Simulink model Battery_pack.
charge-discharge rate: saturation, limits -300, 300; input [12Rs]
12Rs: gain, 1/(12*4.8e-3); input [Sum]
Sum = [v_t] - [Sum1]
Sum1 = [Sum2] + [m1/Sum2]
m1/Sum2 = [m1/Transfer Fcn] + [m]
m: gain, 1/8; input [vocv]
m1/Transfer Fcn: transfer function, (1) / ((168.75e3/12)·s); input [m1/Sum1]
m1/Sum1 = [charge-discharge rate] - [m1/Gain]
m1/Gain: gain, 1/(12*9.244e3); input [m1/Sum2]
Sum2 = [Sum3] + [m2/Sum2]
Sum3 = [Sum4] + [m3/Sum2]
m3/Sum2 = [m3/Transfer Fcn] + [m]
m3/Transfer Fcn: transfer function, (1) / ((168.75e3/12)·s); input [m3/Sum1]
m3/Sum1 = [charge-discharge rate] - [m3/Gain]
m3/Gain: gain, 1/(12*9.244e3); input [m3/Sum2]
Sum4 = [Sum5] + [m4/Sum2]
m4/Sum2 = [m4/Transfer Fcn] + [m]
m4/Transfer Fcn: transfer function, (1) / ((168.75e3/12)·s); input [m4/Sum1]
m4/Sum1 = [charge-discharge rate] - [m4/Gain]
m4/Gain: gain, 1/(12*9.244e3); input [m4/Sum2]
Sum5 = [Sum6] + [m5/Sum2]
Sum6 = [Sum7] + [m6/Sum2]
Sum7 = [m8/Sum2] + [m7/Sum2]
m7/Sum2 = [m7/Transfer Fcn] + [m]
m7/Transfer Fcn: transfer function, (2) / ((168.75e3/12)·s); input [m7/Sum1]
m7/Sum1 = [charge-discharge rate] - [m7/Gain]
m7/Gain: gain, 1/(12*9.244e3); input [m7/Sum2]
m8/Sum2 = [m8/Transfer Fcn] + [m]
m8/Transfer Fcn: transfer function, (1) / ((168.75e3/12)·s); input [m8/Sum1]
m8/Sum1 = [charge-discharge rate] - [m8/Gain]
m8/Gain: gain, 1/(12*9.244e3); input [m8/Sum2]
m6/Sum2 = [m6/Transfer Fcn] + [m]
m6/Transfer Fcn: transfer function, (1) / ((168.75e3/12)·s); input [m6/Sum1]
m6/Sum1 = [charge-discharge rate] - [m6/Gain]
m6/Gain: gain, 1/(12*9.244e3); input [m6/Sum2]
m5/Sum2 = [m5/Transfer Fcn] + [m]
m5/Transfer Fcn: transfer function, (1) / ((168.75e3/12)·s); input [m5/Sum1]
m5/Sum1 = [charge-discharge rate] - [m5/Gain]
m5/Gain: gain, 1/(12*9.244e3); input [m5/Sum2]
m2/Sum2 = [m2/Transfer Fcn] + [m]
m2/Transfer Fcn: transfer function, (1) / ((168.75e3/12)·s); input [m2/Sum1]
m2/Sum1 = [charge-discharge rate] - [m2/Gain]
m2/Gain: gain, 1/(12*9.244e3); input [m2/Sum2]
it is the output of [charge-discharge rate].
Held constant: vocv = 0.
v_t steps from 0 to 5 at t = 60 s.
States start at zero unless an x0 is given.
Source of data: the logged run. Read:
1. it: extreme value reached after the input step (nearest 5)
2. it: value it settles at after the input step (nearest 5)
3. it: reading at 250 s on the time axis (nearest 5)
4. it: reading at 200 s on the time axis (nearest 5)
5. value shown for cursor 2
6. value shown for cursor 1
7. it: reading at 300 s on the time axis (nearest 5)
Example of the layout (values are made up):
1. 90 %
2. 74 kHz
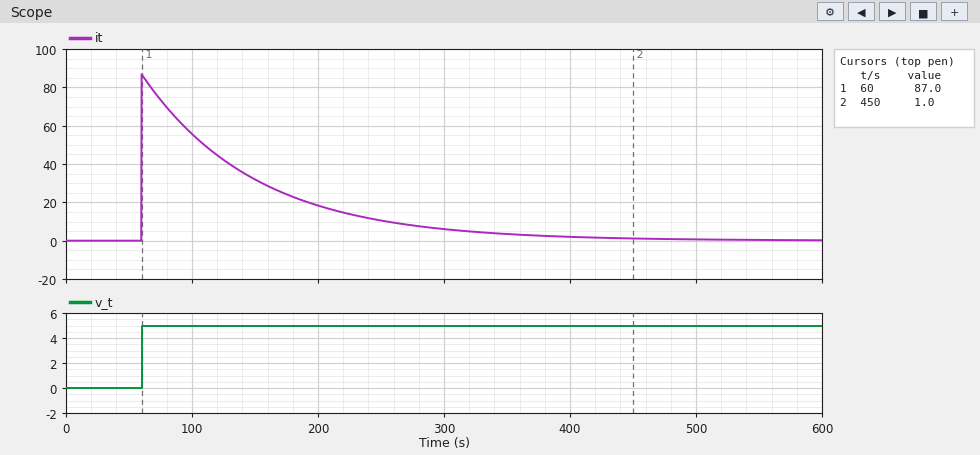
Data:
1. 85
2. 0
3. 10
4. 20
5. 1.0
6. 87.0
7. 5
